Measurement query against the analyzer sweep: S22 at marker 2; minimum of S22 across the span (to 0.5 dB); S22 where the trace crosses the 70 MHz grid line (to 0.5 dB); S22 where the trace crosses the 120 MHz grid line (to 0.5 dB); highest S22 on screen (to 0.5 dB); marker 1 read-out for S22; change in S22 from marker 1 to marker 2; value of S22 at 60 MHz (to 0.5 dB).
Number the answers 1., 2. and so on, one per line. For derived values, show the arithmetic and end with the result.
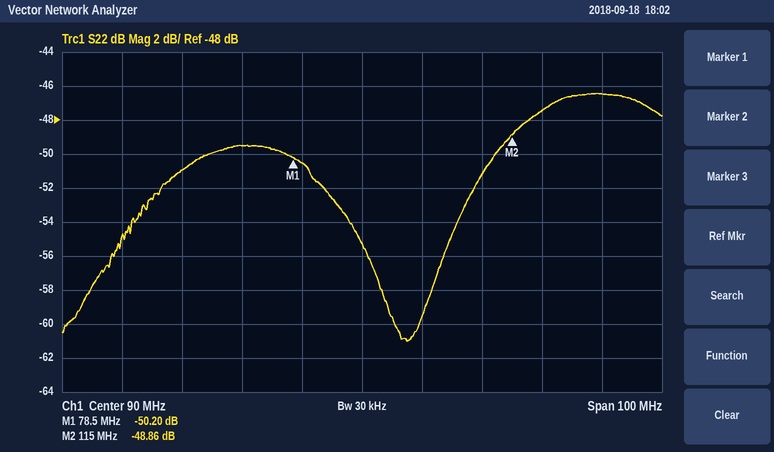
1. -48.86 dB
2. -61.0 dB
3. -49.5 dB
4. -47.5 dB
5. -46.5 dB
6. -50.20 dB
7. -48.86 − (-50.2) = 1.34 dB
8. -51.0 dB
